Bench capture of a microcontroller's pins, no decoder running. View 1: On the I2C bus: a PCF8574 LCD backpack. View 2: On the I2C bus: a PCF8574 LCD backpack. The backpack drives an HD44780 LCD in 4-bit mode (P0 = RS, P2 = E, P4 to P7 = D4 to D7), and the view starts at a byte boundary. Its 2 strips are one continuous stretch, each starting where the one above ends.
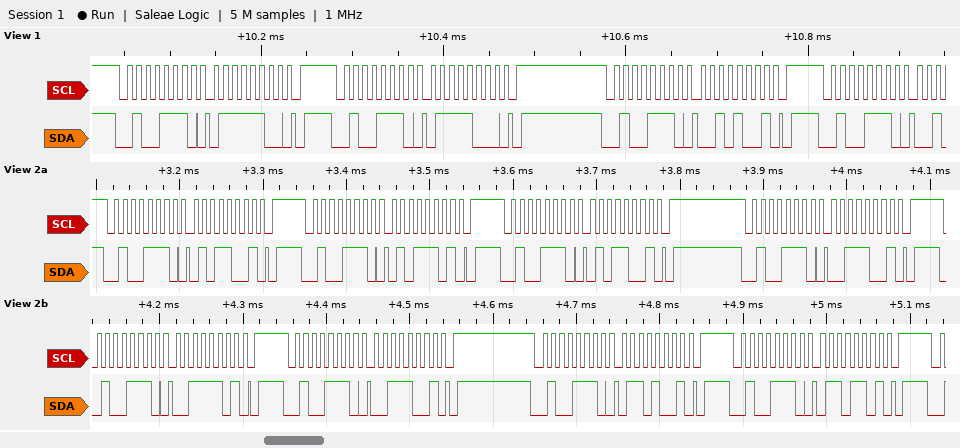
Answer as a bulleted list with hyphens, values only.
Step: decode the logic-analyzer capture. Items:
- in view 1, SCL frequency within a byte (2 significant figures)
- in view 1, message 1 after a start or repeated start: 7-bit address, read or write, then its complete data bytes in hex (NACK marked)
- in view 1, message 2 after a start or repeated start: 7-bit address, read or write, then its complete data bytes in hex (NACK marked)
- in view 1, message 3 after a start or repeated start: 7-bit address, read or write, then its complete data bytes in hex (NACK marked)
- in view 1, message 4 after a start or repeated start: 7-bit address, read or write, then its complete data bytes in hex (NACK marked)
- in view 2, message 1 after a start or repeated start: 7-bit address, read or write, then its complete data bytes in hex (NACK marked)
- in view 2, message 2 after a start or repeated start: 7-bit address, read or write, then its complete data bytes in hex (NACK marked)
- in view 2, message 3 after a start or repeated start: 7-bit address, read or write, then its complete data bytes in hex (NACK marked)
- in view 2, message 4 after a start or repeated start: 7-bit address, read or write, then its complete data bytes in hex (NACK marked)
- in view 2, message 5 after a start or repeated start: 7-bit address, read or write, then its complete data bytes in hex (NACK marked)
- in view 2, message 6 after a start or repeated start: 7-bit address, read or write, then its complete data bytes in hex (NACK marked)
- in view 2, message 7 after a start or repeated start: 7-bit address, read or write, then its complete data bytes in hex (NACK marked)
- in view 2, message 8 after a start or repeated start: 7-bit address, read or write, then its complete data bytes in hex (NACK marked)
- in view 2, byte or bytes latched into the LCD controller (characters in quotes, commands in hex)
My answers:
- 100 kHz
- 0x27 write: 7C
- 0x27 write: 78
- 0x27 write: 29
- 0x27 write
- 0x27 write: 59
- 0x27 write: 5D
- 0x27 write: 59
- 0x27 write: 39
- 0x27 write: 3D
- 0x27 write: 39
- 0x27 write: 69
- 0x27 write: 6D
- 'S'
